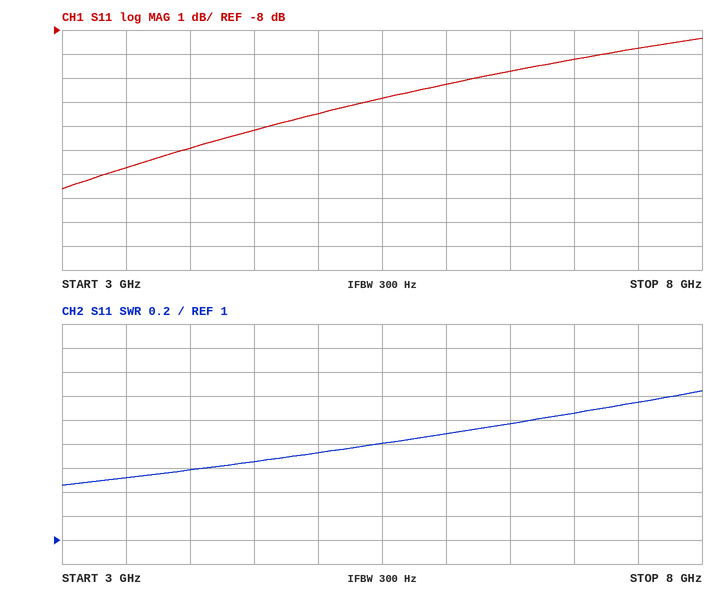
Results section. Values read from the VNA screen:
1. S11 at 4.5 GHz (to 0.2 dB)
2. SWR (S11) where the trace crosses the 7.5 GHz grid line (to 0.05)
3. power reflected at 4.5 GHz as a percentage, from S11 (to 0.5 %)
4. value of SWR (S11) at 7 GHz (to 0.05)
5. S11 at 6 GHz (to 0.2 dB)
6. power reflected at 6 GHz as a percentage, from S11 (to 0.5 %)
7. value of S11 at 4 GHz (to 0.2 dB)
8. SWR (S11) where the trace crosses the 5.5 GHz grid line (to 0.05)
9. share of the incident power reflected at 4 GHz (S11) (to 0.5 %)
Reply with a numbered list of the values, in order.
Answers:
1. -12.2 dB
2. 2.15
3. 6.0 %
4. 2.05
5. -10.2 dB
6. 9.5 %
7. -13.0 dB
8. 1.80
9. 5.0 %
